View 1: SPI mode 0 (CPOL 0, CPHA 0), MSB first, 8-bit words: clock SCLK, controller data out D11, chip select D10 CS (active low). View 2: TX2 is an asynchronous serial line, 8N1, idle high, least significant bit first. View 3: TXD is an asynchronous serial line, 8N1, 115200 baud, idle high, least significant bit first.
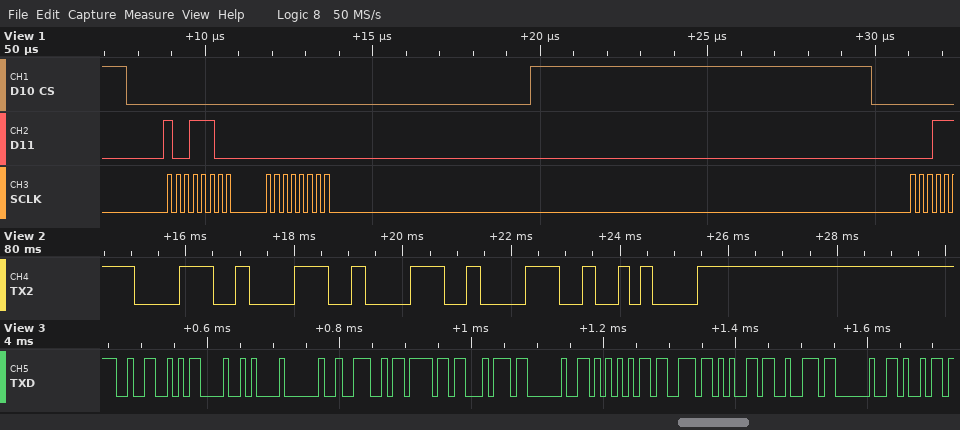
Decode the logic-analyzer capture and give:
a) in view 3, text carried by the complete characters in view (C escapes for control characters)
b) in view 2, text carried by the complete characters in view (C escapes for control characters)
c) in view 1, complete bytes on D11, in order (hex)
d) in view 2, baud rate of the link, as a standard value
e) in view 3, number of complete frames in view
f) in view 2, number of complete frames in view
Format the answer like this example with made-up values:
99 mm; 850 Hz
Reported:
"2\r\n Not User i"; "8888\n"; 9C 00; 4800 baud; 14; 5
